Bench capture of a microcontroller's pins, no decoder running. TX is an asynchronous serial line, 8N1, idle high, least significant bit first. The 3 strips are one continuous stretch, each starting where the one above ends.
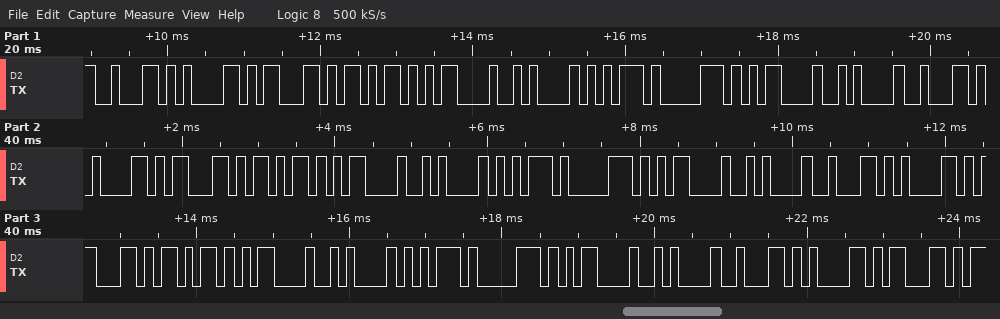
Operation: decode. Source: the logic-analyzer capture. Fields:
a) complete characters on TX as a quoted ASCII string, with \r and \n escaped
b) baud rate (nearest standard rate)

"back\r\nup\r\nback\r\nup\r\nback\r\nup\r\nbac"
9600 baud
